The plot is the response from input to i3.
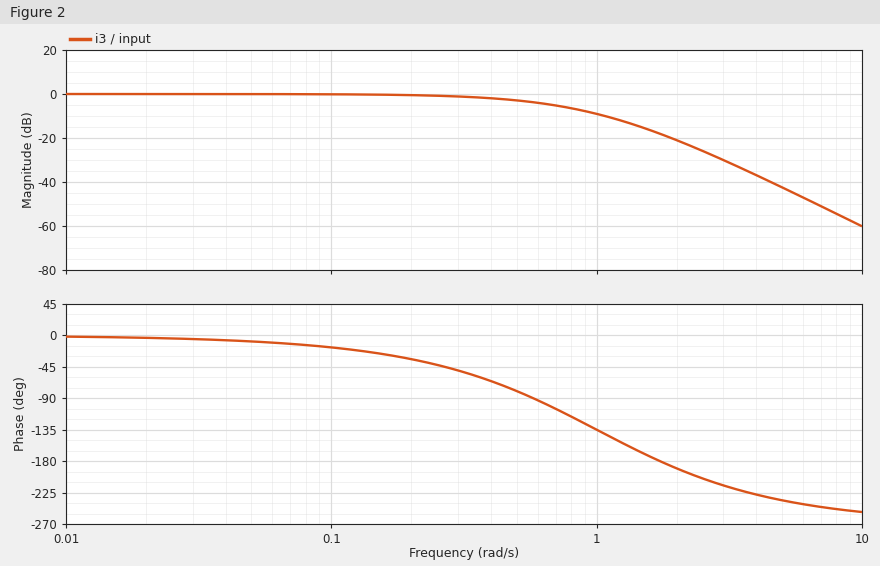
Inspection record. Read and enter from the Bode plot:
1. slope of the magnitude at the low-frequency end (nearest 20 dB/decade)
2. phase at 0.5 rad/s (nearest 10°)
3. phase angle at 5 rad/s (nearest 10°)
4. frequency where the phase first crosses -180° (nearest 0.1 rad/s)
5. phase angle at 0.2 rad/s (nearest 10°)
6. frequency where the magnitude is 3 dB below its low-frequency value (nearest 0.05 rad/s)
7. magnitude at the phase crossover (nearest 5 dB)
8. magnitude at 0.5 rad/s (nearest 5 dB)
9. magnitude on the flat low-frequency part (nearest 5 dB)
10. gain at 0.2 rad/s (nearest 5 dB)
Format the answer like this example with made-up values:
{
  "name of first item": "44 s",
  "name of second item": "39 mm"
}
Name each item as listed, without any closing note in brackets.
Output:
{
  "slope of the magnitude at the low-frequency end": "0 dB/decade",
  "phase at 0.5 rad/s": "-80°",
  "phase angle at 5 rad/s": "-240°",
  "frequency where the phase first crosses -180°": "1.7 rad/s",
  "phase angle at 0.2 rad/s": "-30°",
  "frequency where the magnitude is 3 dB below its low-frequency value": "0.50 rad/s",
  "magnitude at the phase crossover": "-20 dB",
  "magnitude at 0.5 rad/s": "-5 dB",
  "magnitude on the flat low-frequency part": "0 dB",
  "gain at 0.2 rad/s": "0 dB"
}
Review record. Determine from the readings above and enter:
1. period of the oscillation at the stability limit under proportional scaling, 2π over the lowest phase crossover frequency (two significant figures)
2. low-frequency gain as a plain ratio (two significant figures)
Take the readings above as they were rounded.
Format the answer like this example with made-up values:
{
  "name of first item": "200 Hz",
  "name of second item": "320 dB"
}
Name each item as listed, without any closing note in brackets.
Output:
{
  "period of the oscillation at the stability limit under proportional scaling, 2π over the lowest phase crossover frequency": "3.7 s",
  "low-frequency gain as a plain ratio": "1.0"
}
